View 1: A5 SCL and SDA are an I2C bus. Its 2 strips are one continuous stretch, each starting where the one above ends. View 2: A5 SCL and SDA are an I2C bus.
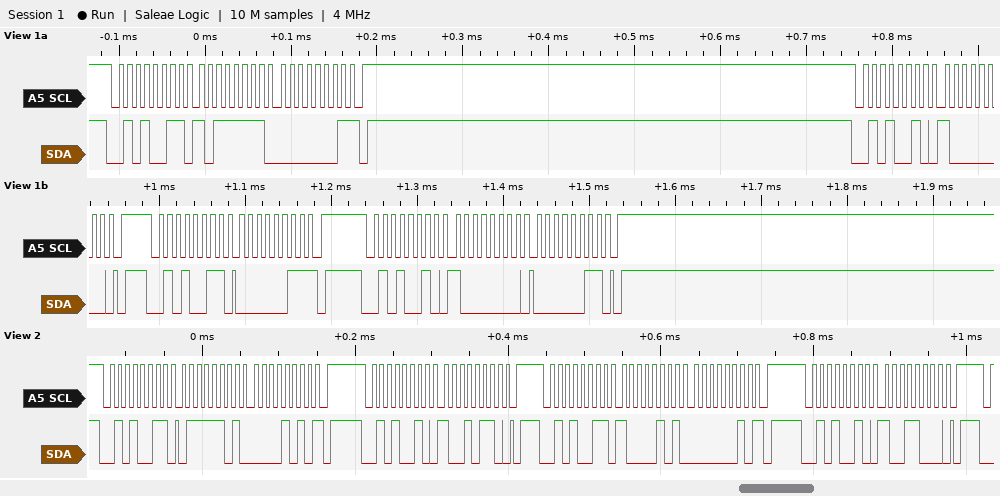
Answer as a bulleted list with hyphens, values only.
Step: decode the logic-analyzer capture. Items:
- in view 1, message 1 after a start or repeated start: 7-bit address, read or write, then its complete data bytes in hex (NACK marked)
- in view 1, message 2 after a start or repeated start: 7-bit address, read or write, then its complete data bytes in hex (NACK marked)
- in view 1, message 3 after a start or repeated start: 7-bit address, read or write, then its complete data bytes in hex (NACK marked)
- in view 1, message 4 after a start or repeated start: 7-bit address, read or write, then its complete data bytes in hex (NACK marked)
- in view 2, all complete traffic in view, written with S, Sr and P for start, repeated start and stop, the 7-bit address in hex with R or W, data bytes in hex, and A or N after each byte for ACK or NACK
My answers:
- 0x29 read: BF 01 NACK
- 0x29 write: 80
- 0x29 read: 03 NACK
- 0x29 write: 80 03
- S 29R A 7D A 0A N P S 29W A 96 A P S 29R A 85 A 02 N P S 29W A 98 A P
